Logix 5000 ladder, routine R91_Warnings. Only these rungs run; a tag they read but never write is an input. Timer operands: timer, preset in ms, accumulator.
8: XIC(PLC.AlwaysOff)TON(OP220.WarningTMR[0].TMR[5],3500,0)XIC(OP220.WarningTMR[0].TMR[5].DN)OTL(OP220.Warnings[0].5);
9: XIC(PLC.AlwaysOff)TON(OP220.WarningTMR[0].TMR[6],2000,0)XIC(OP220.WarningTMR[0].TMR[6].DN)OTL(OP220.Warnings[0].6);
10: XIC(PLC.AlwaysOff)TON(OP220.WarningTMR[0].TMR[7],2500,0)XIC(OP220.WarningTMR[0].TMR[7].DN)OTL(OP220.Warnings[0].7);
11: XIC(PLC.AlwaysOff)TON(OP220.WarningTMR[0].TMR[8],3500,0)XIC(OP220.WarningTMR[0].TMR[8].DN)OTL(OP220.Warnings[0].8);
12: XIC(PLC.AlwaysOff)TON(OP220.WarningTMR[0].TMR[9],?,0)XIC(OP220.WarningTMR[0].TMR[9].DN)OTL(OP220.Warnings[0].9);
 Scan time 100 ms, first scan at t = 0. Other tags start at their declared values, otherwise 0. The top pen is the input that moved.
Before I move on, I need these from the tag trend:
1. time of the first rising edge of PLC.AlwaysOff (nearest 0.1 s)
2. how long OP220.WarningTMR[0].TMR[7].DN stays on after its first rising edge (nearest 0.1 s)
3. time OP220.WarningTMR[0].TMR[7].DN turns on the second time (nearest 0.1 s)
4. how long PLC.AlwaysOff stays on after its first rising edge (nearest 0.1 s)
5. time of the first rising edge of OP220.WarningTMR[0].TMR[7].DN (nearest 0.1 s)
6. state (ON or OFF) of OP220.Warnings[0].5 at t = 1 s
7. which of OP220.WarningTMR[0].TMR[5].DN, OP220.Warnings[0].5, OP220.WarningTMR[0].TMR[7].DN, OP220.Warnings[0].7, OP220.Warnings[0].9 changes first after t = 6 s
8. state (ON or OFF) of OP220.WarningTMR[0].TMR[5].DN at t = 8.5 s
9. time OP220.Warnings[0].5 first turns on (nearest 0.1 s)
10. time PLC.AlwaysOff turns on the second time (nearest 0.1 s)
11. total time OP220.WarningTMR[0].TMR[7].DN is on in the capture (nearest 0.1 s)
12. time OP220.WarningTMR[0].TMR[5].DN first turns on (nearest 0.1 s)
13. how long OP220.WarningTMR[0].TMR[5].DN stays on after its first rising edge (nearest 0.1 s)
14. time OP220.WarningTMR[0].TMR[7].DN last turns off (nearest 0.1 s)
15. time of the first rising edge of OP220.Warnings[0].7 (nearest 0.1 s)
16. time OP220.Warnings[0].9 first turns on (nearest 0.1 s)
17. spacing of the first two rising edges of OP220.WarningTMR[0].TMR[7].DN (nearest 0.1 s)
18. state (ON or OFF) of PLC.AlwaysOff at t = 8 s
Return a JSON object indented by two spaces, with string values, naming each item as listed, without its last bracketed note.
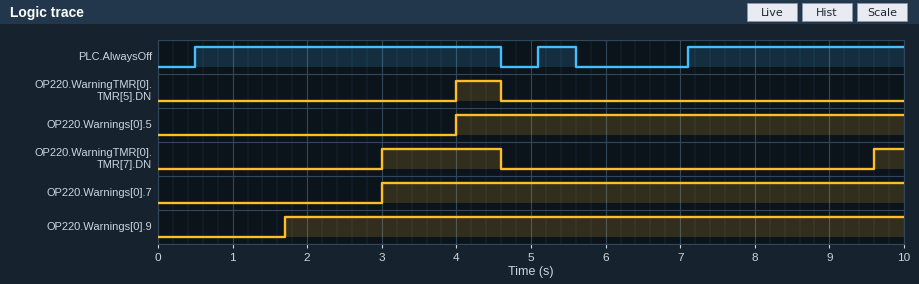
{
  "time of the first rising edge of PLC.AlwaysOff": "0.5 s",
  "how long OP220.WarningTMR[0].TMR[7].DN stays on after its first rising edge": "1.6 s",
  "time OP220.WarningTMR[0].TMR[7].DN turns on the second time": "9.6 s",
  "how long PLC.AlwaysOff stays on after its first rising edge": "4.1 s",
  "time of the first rising edge of OP220.WarningTMR[0].TMR[7].DN": "3.0 s",
  "state (ON or OFF) of OP220.Warnings[0].5 at t = 1 s": "OFF",
  "which of OP220.WarningTMR[0].TMR[5].DN, OP220.Warnings[0].5, OP220.WarningTMR[0].TMR[7].DN, OP220.Warnings[0].7, OP220.Warnings[0].9 changes first after t = 6 s": "OP220.WarningTMR[0].TMR[7].DN",
  "state (ON or OFF) of OP220.WarningTMR[0].TMR[5].DN at t = 8.5 s": "OFF",
  "time OP220.Warnings[0].5 first turns on": "4.0 s",
  "time PLC.AlwaysOff turns on the second time": "5.1 s",
  "total time OP220.WarningTMR[0].TMR[7].DN is on in the capture": "2.0 s",
  "time OP220.WarningTMR[0].TMR[5].DN first turns on": "4.0 s",
  "how long OP220.WarningTMR[0].TMR[5].DN stays on after its first rising edge": "0.6 s",
  "time OP220.WarningTMR[0].TMR[7].DN last turns off": "4.6 s",
  "time of the first rising edge of OP220.Warnings[0].7": "3.0 s",
  "time OP220.Warnings[0].9 first turns on": "1.7 s",
  "spacing of the first two rising edges of OP220.WarningTMR[0].TMR[7].DN": "6.6 s",
  "state (ON or OFF) of PLC.AlwaysOff at t = 8 s": "ON"
}
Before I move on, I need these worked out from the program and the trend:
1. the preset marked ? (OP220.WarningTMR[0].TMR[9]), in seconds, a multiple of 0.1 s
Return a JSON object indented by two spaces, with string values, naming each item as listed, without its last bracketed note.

{
  "the preset marked ? (OP220.WarningTMR[0].TMR[9]), in seconds, a multiple of 0.1 s": "1.2 s"
}
